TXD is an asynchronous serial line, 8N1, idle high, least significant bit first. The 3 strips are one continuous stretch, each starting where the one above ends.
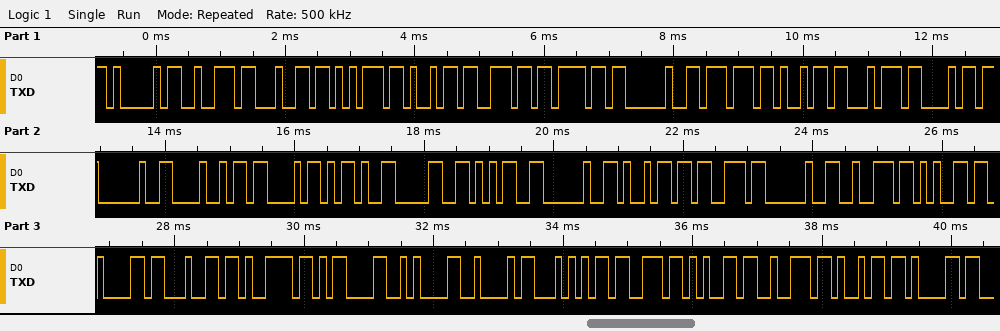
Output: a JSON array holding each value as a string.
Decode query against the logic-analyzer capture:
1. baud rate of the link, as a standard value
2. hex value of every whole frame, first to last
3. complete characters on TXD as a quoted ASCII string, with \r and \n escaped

["9600 baud", "41 72 64 75 69 6E 6F 20 77 69 74 68 20 48 43 2D 30 35 20 69 73 20 72 65 61 64 79 0D 0A 42 54 73 65 72 69 61", "\"Arduino with HC-05 is ready\\r\\nBTseria\""]
